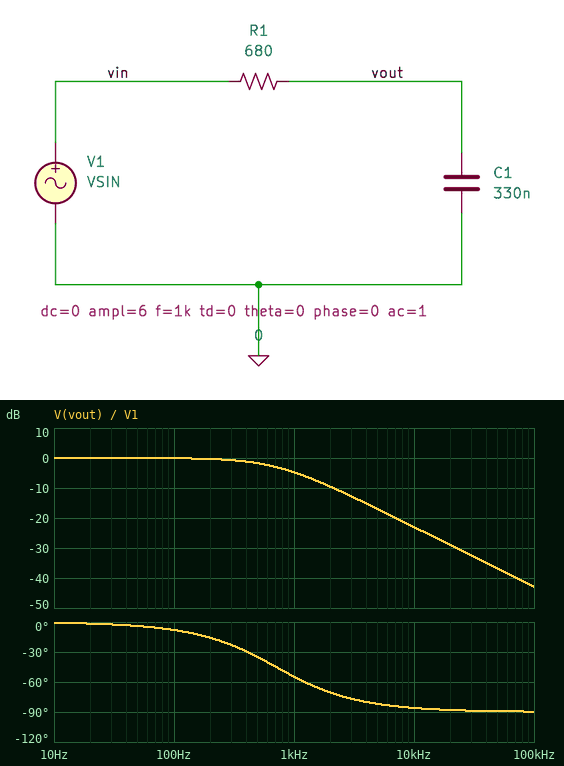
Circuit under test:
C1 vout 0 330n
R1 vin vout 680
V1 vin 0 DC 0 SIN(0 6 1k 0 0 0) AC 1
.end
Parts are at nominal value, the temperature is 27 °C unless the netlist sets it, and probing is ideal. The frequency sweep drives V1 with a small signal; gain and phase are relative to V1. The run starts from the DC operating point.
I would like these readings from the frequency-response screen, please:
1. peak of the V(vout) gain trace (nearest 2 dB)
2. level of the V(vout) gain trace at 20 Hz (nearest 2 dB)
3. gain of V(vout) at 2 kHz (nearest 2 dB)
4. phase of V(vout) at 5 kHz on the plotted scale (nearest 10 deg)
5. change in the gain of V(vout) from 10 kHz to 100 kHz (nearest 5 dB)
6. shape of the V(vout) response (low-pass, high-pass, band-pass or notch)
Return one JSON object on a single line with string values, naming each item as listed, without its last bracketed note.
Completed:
{"peak of the V(vout) gain trace": "0 dB", "level of the V(vout) gain trace at 20 Hz": "0 dB", "gain of V(vout) at 2 kHz": "-10 dB", "phase of V(vout) at 5 kHz on the plotted scale": "-80 deg", "change in the gain of V(vout) from 10 kHz to 100 kHz": "-20 dB", "shape of the V(vout) response": "low-pass"}
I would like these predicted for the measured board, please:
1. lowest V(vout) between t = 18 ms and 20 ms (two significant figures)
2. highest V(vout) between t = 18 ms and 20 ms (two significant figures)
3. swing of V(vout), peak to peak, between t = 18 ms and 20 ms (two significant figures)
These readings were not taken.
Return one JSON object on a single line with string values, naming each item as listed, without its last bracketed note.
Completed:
{"lowest V(vout) between t = 18 ms and 20 ms": "-3.5 V", "highest V(vout) between t = 18 ms and 20 ms": "3.5 V", "swing of V(vout), peak to peak, between t = 18 ms and 20 ms": "6.9 V"}
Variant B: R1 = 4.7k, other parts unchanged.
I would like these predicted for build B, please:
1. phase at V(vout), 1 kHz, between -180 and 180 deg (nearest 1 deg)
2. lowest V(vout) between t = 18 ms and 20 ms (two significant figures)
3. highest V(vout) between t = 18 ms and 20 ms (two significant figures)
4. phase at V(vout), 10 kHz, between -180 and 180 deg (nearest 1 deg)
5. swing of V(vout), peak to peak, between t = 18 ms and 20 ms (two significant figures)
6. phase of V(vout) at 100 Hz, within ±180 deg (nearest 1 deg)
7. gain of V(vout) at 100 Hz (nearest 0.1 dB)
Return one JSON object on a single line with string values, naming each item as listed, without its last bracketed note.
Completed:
{"phase at V(vout), 1 kHz, between -180 and 180 deg": "-84 deg", "lowest V(vout) between t = 18 ms and 20 ms": "-610 mV", "highest V(vout) between t = 18 ms and 20 ms": "610 mV", "phase at V(vout), 10 kHz, between -180 and 180 deg": "-89 deg", "swing of V(vout), peak to peak, between t = 18 ms and 20 ms": "1.2 V", "phase of V(vout) at 100 Hz, within ±180 deg": "-44 deg", "gain of V(vout) at 100 Hz": "-2.9 dB"}
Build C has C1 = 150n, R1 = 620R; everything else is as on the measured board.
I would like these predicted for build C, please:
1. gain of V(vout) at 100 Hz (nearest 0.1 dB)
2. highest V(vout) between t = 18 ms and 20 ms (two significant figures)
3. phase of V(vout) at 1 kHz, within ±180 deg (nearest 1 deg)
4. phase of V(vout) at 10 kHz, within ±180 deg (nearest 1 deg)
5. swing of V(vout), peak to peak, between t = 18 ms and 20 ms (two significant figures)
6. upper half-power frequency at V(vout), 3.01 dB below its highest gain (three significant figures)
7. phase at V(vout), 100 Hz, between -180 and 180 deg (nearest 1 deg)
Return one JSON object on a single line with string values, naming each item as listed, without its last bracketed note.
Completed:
{"gain of V(vout) at 100 Hz": "0 dB", "highest V(vout) between t = 18 ms and 20 ms": "5.2 V", "phase of V(vout) at 1 kHz, within ±180 deg": "-30 deg", "phase of V(vout) at 10 kHz, within ±180 deg": "-80 deg", "swing of V(vout), peak to peak, between t = 18 ms and 20 ms": "10 V", "upper half-power frequency at V(vout), 3.01 dB below its highest gain": "1.71 kHz", "phase at V(vout), 100 Hz, between -180 and 180 deg": "-3 deg"}
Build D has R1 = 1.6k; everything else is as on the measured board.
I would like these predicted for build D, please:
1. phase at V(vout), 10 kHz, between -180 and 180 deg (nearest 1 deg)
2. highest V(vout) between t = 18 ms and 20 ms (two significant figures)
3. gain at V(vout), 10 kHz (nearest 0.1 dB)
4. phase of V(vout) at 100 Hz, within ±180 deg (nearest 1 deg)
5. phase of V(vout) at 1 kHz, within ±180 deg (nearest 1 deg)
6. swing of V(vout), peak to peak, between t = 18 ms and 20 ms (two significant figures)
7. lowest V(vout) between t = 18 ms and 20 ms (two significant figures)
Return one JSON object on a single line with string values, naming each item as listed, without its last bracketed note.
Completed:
{"phase at V(vout), 10 kHz, between -180 and 180 deg": "-88 deg", "highest V(vout) between t = 18 ms and 20 ms": "1.7 V", "gain at V(vout), 10 kHz": "-30.4 dB", "phase of V(vout) at 100 Hz, within ±180 deg": "-18 deg", "phase of V(vout) at 1 kHz, within ±180 deg": "-73 deg", "swing of V(vout), peak to peak, between t = 18 ms and 20 ms": "3.5 V", "lowest V(vout) between t = 18 ms and 20 ms": "-1.7 V"}
